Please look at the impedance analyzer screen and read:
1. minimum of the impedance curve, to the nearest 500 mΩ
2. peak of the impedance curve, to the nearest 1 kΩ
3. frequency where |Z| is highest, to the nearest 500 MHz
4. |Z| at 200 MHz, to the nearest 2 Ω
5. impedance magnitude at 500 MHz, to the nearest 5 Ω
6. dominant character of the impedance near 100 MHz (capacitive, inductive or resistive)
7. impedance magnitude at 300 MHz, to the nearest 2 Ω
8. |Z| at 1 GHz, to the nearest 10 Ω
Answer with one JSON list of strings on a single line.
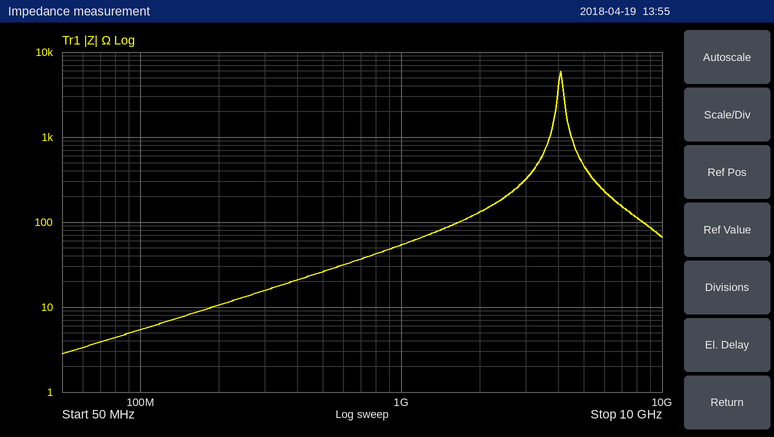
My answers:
["3.0 Ω", "6 kΩ", "4.0 GHz", "10 Ω", "25 Ω", "inductive", "16 Ω", "50 Ω"]
